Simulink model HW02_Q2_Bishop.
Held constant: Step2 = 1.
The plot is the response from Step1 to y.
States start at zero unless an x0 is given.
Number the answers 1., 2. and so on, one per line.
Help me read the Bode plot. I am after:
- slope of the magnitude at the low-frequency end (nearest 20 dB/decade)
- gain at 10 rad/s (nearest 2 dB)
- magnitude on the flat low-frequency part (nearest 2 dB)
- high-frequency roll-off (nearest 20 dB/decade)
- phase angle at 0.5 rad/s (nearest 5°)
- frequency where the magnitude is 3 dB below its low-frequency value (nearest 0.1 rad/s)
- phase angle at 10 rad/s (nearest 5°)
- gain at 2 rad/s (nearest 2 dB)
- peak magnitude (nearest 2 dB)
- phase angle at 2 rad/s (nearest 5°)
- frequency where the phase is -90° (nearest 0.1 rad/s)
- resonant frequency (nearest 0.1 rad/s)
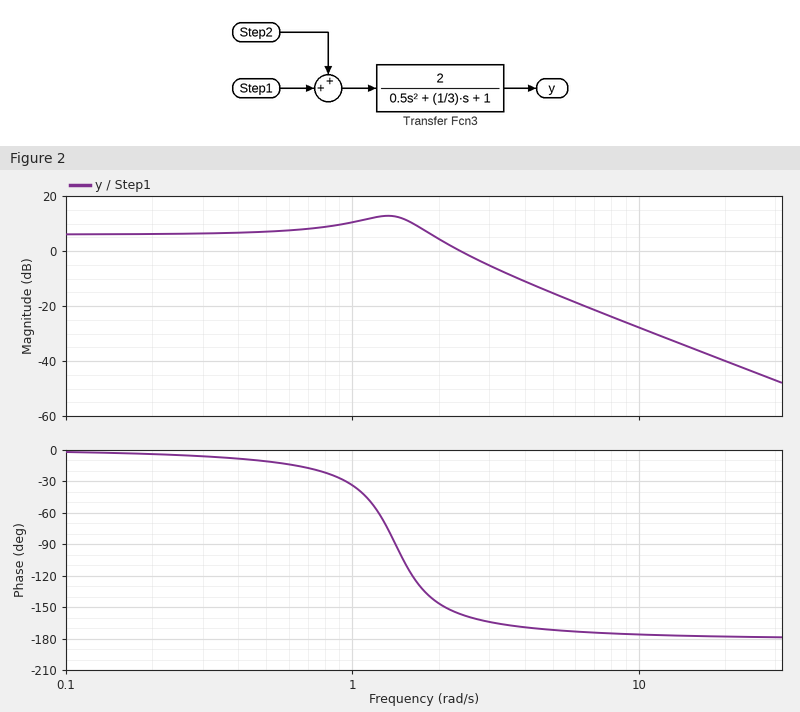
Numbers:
1. 0 dB/decade
2. -28 dB
3. 6 dB
4. -40 dB/decade
5. -10°
6. 2.1 rad/s
7. -175°
8. 4 dB
9. 12 dB
10. -145°
11. 1.4 rad/s
12. 1.3 rad/s
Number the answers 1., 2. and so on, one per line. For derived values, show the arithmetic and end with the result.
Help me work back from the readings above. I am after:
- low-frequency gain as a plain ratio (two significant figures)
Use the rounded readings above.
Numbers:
1. 10^(6 / 20) = 2.0
